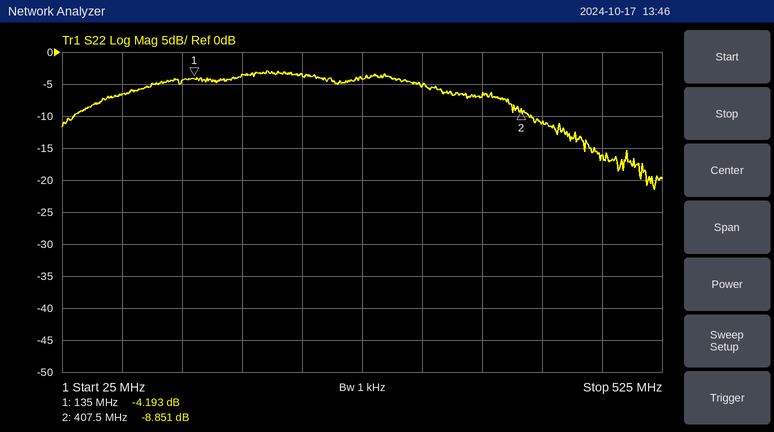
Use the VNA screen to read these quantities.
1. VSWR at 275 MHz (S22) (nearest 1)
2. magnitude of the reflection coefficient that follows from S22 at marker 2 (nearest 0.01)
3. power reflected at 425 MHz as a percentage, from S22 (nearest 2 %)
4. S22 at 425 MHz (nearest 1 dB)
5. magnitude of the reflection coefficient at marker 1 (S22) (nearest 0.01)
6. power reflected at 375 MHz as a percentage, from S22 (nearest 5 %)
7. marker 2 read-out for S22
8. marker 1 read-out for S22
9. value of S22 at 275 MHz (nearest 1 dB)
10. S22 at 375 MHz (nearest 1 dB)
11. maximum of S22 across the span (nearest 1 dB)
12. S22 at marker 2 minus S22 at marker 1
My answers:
4
0.36
8 %
-11 dB
0.62
20 %
-8.851 dB
-4.193 dB
-4 dB
-7 dB
-3 dB
-4.658 dB
